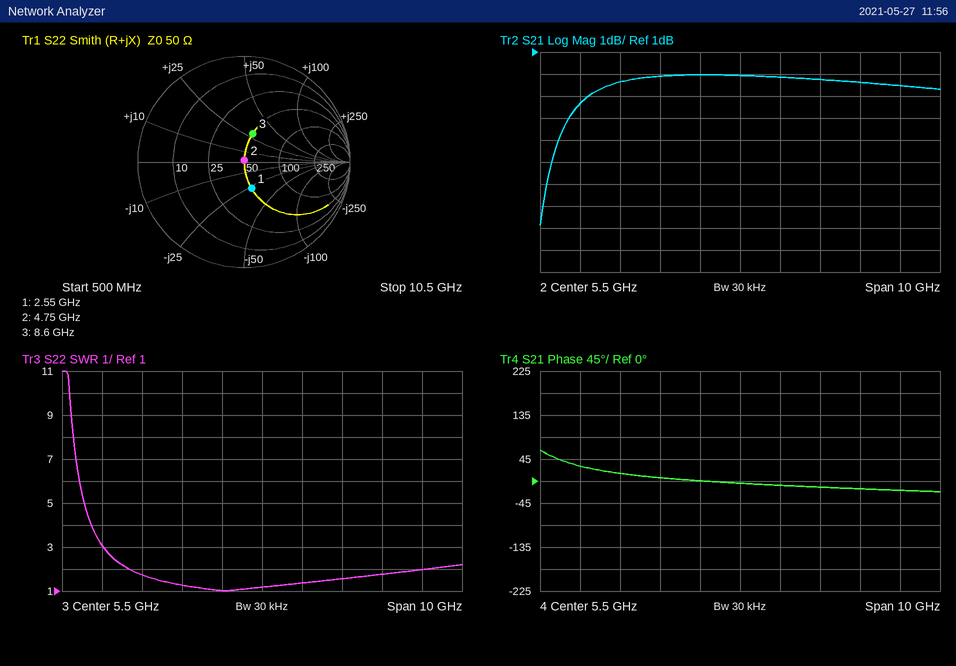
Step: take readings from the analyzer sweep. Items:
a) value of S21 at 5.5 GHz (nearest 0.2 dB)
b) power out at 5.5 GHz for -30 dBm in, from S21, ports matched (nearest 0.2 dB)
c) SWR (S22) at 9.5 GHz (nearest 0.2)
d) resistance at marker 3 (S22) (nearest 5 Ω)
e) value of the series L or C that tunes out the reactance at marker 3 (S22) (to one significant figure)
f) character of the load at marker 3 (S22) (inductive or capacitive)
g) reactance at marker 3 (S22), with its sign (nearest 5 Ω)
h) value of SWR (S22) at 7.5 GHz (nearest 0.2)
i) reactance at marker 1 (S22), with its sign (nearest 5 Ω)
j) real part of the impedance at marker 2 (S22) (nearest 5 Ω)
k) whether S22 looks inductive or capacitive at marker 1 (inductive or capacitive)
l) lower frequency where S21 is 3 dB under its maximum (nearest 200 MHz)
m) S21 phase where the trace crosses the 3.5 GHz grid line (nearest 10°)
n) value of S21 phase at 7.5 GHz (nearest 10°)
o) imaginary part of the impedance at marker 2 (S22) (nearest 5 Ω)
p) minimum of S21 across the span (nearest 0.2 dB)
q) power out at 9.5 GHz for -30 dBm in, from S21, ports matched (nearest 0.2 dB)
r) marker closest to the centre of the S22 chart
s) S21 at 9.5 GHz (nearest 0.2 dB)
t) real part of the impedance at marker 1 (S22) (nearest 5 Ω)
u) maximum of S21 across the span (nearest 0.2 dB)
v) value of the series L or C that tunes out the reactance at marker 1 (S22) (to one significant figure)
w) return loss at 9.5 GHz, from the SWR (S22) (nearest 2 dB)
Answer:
0.0 dB
-30.0 dBm
2.0
50 Ω
600 fF
inductive
+30 Ω
1.6
-25 Ω
50 Ω
capacitive
1.0 GHz
10°
-10°
0 Ω
-6.8 dB
-30.6 dBm
marker 2
-0.6 dB
50 Ω
0.0 dB
2 nH
10 dB
